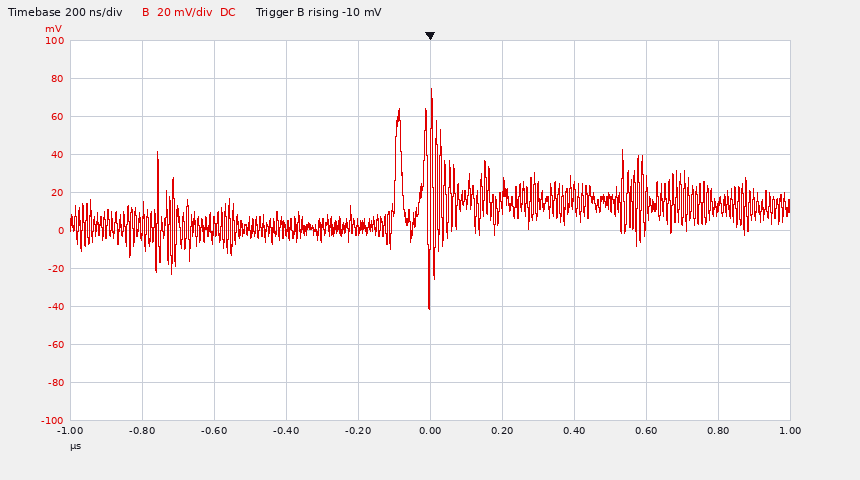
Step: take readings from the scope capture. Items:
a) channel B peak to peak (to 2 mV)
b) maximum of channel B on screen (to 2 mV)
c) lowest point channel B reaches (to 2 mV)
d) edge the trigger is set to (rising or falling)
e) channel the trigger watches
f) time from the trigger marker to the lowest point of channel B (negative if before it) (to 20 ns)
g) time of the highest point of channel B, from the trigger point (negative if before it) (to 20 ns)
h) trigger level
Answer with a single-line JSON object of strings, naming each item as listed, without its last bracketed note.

{"channel B peak to peak": "116 mV", "maximum of channel B on screen": "74 mV", "lowest point channel B reaches": "-42 mV", "edge the trigger is set to": "rising", "channel the trigger watches": "channel B", "time from the trigger marker to the lowest point of channel B (negative if before it)": "0 ns", "time of the highest point of channel B, from the trigger point (negative if before it)": "0 ns", "trigger level": "-10 mV"}
